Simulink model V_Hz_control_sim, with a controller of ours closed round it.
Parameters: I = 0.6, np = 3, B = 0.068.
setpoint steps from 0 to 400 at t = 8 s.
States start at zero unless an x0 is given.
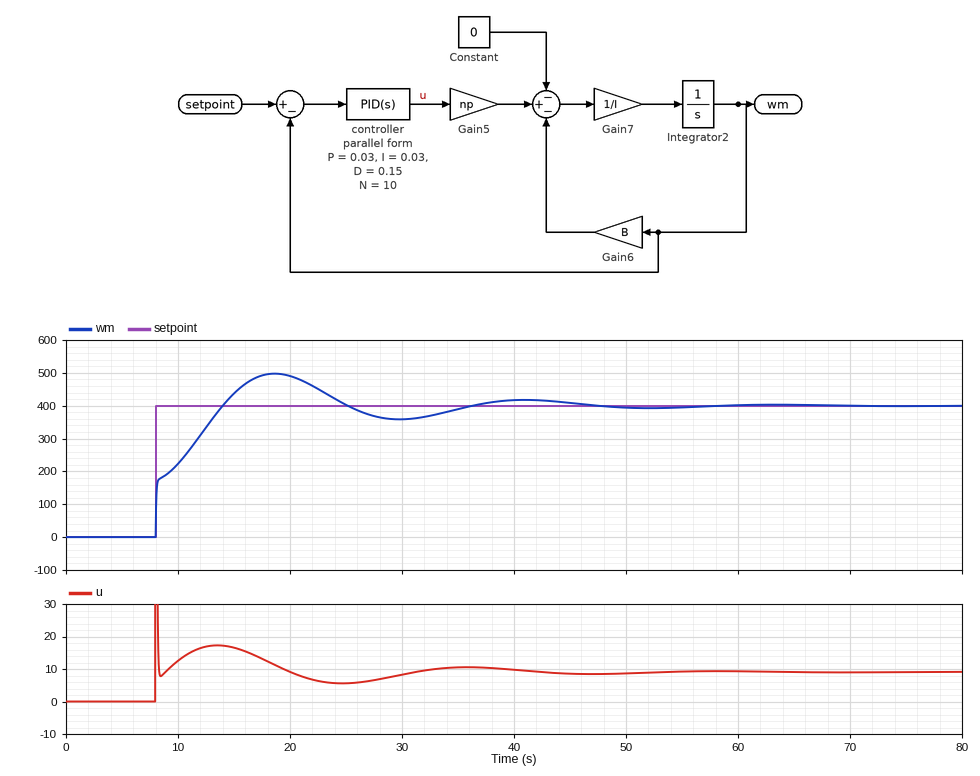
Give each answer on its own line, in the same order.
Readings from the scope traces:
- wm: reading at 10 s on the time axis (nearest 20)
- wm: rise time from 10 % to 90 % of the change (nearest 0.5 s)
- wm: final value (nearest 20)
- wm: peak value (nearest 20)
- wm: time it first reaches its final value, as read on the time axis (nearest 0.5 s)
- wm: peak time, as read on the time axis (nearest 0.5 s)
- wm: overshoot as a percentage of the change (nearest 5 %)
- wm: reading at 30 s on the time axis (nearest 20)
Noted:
220
5.0 s
400
500
14.0 s
18.5 s
25 %
360
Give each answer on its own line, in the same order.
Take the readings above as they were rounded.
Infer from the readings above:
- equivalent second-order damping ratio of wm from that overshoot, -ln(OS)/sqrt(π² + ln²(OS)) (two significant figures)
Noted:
0.40
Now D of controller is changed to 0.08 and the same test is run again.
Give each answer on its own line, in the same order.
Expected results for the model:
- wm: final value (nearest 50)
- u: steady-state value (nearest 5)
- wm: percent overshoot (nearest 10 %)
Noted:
400
10
30 %
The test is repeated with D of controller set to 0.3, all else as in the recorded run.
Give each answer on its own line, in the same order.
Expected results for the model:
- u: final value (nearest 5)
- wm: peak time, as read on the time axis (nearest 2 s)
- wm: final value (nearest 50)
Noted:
10
22 s
400
